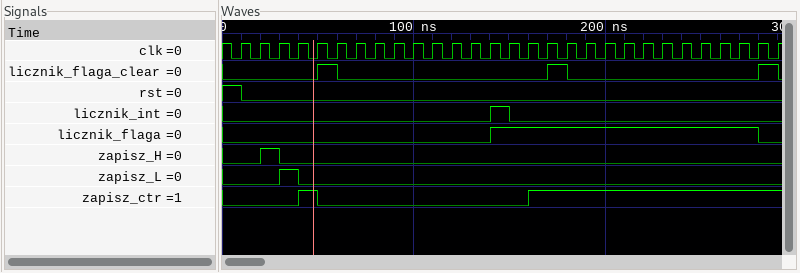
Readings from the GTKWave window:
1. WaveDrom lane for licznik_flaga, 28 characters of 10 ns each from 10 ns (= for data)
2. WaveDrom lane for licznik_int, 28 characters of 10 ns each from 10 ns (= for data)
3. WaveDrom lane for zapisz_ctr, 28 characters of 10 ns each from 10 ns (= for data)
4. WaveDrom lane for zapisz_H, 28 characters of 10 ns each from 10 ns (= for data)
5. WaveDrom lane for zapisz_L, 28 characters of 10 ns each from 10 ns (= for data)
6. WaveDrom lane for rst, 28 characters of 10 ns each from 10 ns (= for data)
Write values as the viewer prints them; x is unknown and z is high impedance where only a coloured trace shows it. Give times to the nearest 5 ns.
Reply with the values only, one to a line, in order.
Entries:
{name: 'licznik_flaga', wave: '0............1.............0'}
{name: 'licznik_int', wave: '0............10.............'}
{name: 'zapisz_ctr', wave: '0..10..........1............'}
{name: 'zapisz_H', wave: '010.........................'}
{name: 'zapisz_L', wave: '0.10........................'}
{name: 'rst', wave: '0...........................'}
